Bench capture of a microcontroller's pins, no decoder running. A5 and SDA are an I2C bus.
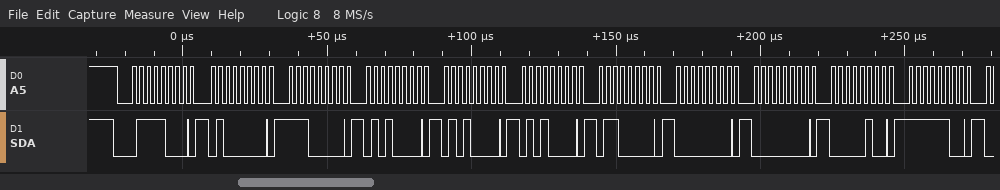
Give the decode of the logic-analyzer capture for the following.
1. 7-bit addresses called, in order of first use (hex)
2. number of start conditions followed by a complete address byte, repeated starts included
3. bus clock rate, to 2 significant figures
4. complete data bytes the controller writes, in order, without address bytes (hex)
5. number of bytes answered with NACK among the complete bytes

0x3C
1
400 kHz
40 E0 50 50 50 60 00 00 04 FC
0
